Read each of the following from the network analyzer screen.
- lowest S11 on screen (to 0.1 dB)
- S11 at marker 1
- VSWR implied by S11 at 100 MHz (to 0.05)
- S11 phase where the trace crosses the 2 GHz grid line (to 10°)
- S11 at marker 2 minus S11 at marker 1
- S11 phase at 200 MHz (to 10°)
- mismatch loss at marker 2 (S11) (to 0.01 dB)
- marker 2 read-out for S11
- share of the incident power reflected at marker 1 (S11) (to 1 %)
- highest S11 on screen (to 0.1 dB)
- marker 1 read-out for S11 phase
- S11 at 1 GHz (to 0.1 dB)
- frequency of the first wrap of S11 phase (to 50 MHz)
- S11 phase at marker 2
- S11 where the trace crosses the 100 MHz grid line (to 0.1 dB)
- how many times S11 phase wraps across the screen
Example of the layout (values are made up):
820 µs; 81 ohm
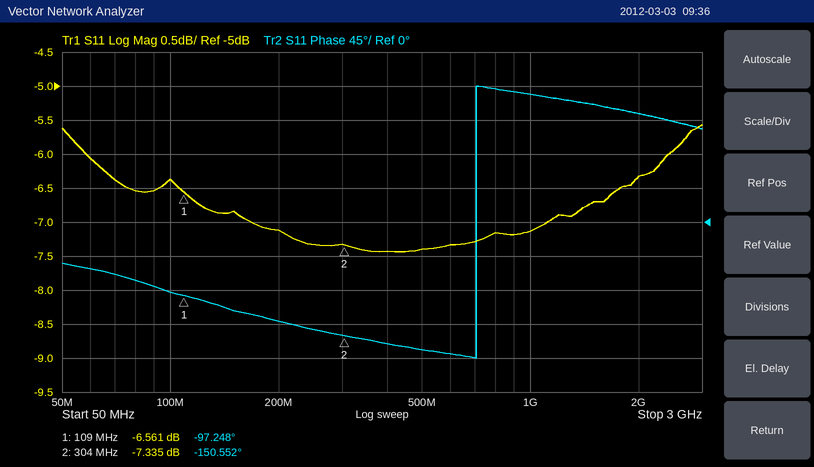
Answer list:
-7.4 dB; -6.561 dB; 2.85; 140°; -0.774 dB; -130°; 0.89 dB; -7.335 dB; 22 %; -5.6 dB; -97.248°; -7.1 dB; 700 MHz; -150.552°; -6.4 dB; 1
